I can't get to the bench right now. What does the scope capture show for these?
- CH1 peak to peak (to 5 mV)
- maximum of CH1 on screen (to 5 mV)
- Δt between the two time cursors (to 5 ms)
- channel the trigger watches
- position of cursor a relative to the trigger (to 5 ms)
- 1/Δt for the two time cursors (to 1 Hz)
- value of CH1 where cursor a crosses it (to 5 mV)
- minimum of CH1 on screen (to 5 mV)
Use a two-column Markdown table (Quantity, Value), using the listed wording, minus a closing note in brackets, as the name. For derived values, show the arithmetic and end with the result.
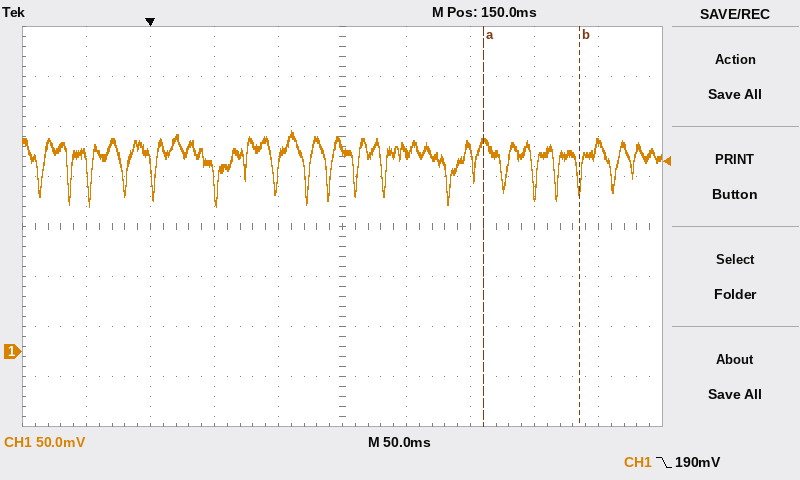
| Quantity | Value |
|---|---|
| CH1 peak to peak | 220 mV − (145 mV) = 75 mV |
| maximum of CH1 on screen | 220 mV |
| Δt between the two time cursors | 75 ms |
| channel the trigger watches | CH1 |
| position of cursor a relative to the trigger | +260 ms |
| 1/Δt for the two time cursors | 1 / 75 ms ≈ 13 Hz |
| value of CH1 where cursor a crosses it | 210 mV |
| minimum of CH1 on screen | 145 mV |
